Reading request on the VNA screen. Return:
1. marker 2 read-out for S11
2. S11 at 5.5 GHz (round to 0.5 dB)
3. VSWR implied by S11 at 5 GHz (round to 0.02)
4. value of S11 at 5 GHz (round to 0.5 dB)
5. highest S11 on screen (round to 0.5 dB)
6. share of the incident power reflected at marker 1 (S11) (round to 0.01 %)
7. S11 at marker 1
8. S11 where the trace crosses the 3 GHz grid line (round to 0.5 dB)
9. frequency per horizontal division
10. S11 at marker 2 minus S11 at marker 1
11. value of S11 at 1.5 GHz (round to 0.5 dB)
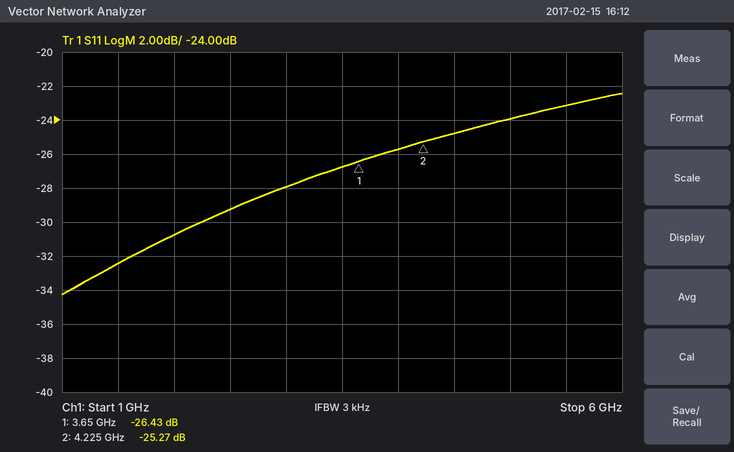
-25.27 dB
-23.0 dB
1.14
-24.0 dB
-22.5 dB
0.23 %
-26.43 dB
-28.0 dB
500 MHz
1.16 dB
-32.5 dB
